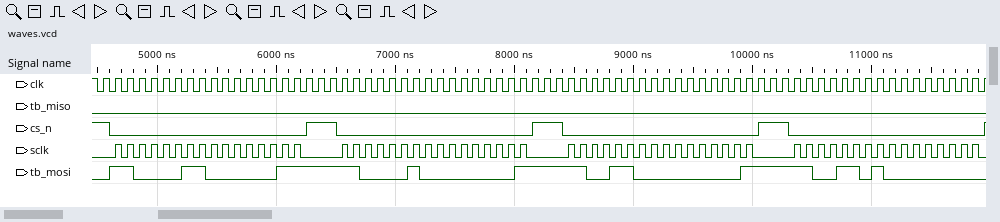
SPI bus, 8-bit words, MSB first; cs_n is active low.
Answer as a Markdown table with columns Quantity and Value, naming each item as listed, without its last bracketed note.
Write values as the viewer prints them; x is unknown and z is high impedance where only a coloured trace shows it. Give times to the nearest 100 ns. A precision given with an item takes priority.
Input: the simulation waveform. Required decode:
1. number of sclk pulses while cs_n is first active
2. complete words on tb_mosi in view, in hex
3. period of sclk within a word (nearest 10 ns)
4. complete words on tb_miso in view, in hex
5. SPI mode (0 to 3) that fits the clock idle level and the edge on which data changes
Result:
| Quantity | Value |
|---|---|
| number of sclk pulses while cs_n is first active | 16 |
| complete words on tb_mosi in view, in hex | C3, 03, C2, 01, CC, 01, CD, 00 |
| period of sclk within a word | 100 ns |
| complete words on tb_miso in view, in hex | 00, 00, 00, 00, 00, 00, 00, 00 |
| SPI mode (0 to 3) that fits the clock idle level and the edge on which data changes | 0 |
